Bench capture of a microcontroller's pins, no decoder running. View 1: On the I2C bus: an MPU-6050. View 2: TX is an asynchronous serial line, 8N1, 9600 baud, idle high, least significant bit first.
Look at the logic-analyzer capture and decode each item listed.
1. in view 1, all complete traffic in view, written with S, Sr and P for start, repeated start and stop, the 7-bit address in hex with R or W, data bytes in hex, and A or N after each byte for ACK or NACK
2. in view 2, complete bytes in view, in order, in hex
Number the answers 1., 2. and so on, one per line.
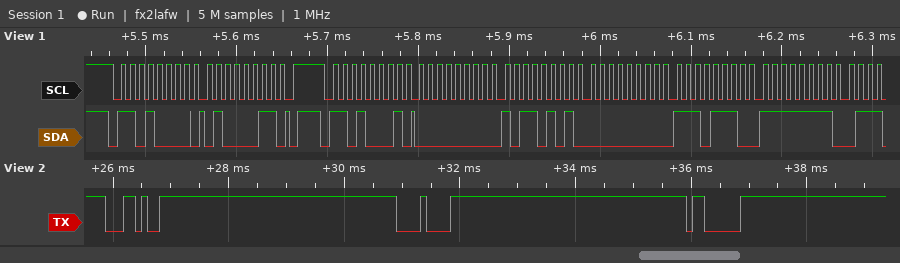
1. S 68W A 43 A P S 68R A 00 A B5 A 00 A EE A FF A
2. 0x2C 0x08 0x03
